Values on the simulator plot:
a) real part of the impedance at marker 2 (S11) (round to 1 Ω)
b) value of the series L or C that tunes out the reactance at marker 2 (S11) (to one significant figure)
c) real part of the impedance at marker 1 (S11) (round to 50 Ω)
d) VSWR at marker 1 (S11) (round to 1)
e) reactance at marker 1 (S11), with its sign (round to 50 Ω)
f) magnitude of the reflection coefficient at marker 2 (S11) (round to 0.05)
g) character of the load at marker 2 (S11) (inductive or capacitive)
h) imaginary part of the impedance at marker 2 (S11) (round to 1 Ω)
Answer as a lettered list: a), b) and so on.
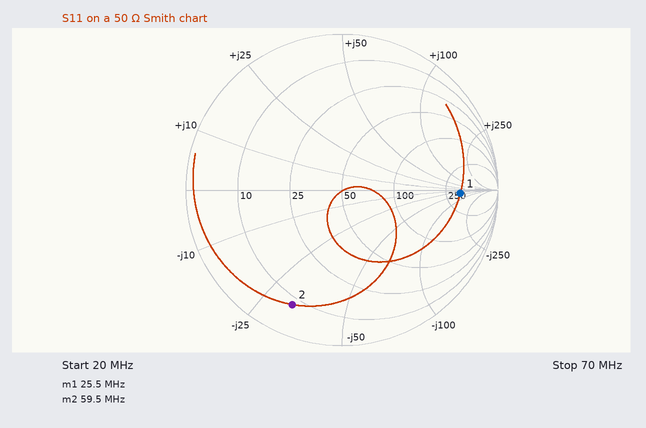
a) 8 Ω
b) 90 nH
c) 350 Ω
d) 7
e) -50 Ω
f) 0.80
g) capacitive
h) -32 Ω
